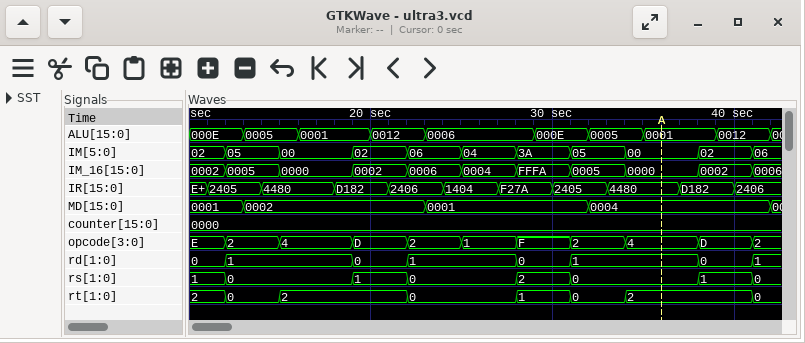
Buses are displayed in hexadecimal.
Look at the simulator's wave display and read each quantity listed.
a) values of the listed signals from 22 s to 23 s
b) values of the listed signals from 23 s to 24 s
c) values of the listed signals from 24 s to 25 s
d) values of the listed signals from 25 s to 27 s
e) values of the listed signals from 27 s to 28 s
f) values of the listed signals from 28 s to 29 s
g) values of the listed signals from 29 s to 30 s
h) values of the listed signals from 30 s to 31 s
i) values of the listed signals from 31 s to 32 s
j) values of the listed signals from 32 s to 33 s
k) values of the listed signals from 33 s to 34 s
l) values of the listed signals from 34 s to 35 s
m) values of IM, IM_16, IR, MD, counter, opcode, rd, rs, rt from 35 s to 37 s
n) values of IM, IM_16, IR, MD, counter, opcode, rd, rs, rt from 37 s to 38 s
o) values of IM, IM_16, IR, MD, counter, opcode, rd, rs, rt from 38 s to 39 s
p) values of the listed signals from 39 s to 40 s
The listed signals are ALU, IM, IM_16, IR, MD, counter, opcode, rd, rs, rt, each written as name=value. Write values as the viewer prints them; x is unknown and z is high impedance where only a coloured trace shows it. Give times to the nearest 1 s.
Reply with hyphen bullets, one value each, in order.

- ALU=0012, IM=06, IM_16=0006, IR=2406, MD=0002, counter=0000, opcode=2, rd=1, rs=0, rt=0
- ALU=0006, IM=06, IM_16=0006, IR=2406, MD=0001, counter=0000, opcode=2, rd=1, rs=0, rt=0
- ALU=0006, IM=06, IM_16=0006, IR=1404, MD=0001, counter=0000, opcode=2, rd=1, rs=0, rt=0
- ALU=0006, IM=04, IM_16=0004, IR=1404, MD=0001, counter=0000, opcode=1, rd=1, rs=0, rt=0
- ALU=0006, IM=04, IM_16=0004, IR=F27A, MD=0001, counter=0000, opcode=1, rd=1, rs=0, rt=0
- ALU=0006, IM=3A, IM_16=FFFA, IR=F27A, MD=0001, counter=0000, opcode=F, rd=0, rs=2, rt=1
- ALU=000E, IM=3A, IM_16=FFFA, IR=F27A, MD=0001, counter=0000, opcode=F, rd=0, rs=2, rt=1
- ALU=000E, IM=3A, IM_16=FFFA, IR=2405, MD=0001, counter=0000, opcode=F, rd=0, rs=2, rt=1
- ALU=000E, IM=05, IM_16=0005, IR=2405, MD=0001, counter=0000, opcode=2, rd=1, rs=0, rt=0
- ALU=0005, IM=05, IM_16=0005, IR=2405, MD=0004, counter=0000, opcode=2, rd=1, rs=0, rt=0
- ALU=0005, IM=05, IM_16=0005, IR=4480, MD=0004, counter=0000, opcode=2, rd=1, rs=0, rt=0
- ALU=0005, IM=00, IM_16=0000, IR=4480, MD=0004, counter=0000, opcode=4, rd=1, rs=0, rt=2
- IM=00, IM_16=0000, IR=4480, MD=0004, counter=0000, opcode=4, rd=1, rs=0, rt=2
- IM=00, IM_16=0000, IR=D182, MD=0004, counter=0000, opcode=4, rd=1, rs=0, rt=2
- IM=02, IM_16=0002, IR=D182, MD=0004, counter=0000, opcode=D, rd=0, rs=1, rt=2
- ALU=0012, IM=02, IM_16=0002, IR=D182, MD=0004, counter=0000, opcode=D, rd=0, rs=1, rt=2
